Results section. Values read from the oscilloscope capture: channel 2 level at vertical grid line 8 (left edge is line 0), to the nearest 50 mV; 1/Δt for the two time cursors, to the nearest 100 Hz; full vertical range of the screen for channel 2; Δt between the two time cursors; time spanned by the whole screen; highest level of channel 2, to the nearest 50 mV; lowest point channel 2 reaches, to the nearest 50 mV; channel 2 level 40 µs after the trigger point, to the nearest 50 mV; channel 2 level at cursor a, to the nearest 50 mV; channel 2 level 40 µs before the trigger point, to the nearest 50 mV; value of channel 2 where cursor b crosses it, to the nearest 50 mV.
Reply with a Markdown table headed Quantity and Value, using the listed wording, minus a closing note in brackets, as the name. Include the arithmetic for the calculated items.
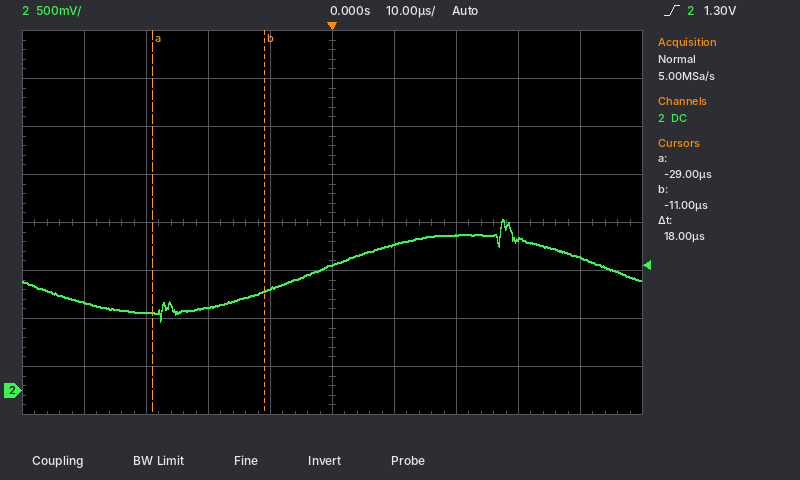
| Quantity | Value |
|---|---|
| channel 2 level at vertical grid line 8 (left edge is line 0), to the nearest 50 mV | 1.55 V |
| 1/Δt for the two time cursors, to the nearest 100 Hz | 1 / 18 µs ≈ 55.6 kHz |
| full vertical range of the screen for channel 2 | 4 V |
| Δt between the two time cursors | 18 µs |
| time spanned by the whole screen | 100 µs |
| highest level of channel 2, to the nearest 50 mV | 1.80 V |
| lowest point channel 2 reaches, to the nearest 50 mV | 700 mV |
| channel 2 level 40 µs after the trigger point, to the nearest 50 mV | 1.40 V |
| channel 2 level at cursor a, to the nearest 50 mV | 800 mV |
| channel 2 level 40 µs before the trigger point, to the nearest 50 mV | 900 mV |
| value of channel 2 where cursor b crosses it, to the nearest 50 mV | 1.05 V |
